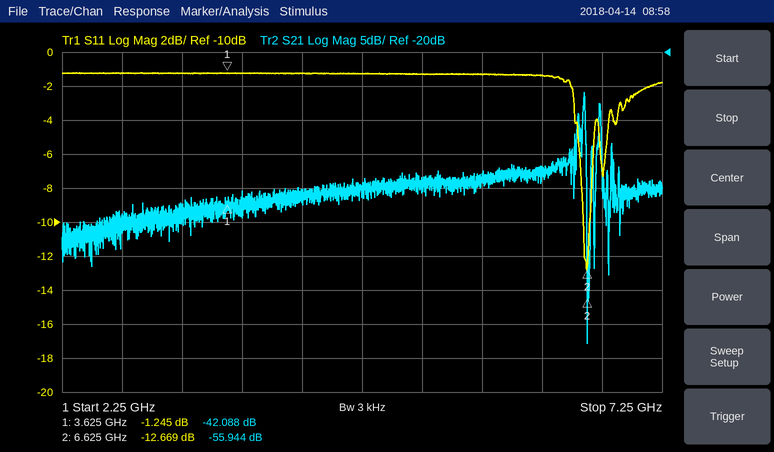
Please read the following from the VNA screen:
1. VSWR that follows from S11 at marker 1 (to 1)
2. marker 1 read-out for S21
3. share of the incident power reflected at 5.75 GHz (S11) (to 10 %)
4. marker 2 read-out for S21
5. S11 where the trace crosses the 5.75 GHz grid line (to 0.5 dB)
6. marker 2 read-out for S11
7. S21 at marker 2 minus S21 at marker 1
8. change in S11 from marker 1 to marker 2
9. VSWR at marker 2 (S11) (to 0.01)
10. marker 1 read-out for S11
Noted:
14
-42.088 dB
70 %
-55.944 dB
-1.5 dB
-12.669 dB
-13.856 dB
-11.424 dB
1.61
-1.245 dB
